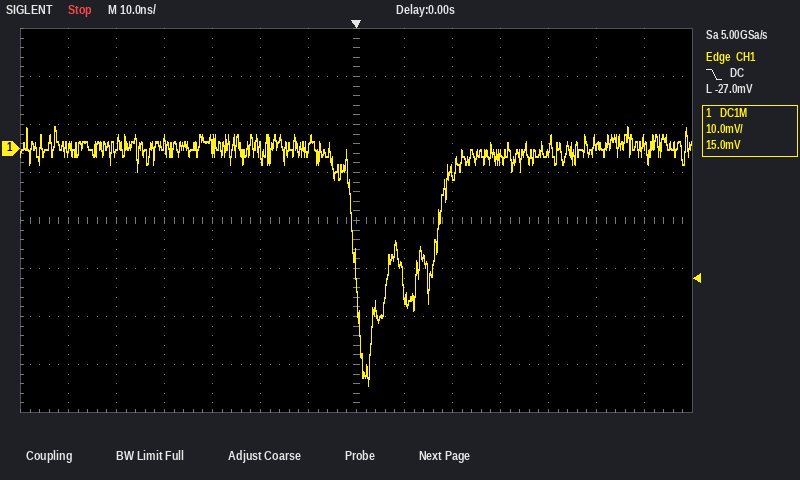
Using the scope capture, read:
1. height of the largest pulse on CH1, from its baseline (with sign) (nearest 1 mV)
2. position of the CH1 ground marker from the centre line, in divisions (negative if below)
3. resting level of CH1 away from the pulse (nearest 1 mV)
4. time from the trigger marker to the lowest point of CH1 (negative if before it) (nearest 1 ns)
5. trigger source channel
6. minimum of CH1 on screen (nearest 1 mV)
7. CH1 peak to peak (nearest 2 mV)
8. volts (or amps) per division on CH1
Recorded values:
-49 mV
+1.5 div
0 mV
+3 ns
CH1
-49 mV
54 mV
10 mV
